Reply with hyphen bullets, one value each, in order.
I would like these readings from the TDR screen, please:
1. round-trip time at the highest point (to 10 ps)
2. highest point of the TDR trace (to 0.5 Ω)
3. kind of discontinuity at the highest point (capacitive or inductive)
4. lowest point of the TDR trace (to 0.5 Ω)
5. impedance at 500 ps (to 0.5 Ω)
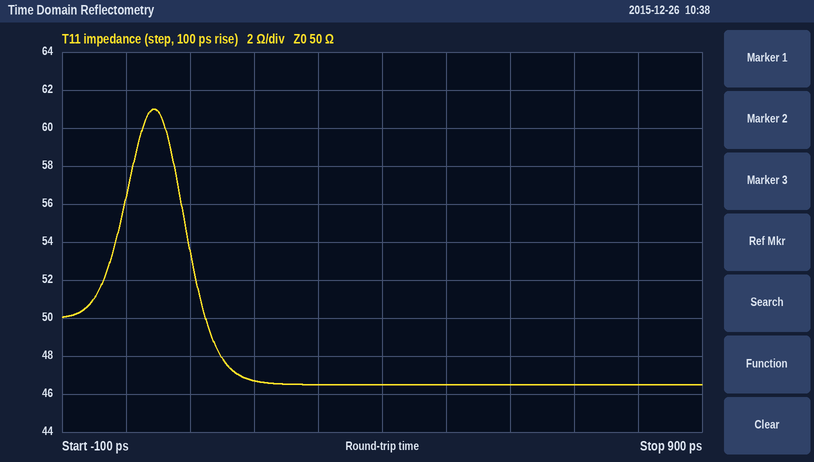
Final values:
- 40 ps
- 61.0 Ω
- inductive
- 46.5 Ω
- 46.5 Ω
